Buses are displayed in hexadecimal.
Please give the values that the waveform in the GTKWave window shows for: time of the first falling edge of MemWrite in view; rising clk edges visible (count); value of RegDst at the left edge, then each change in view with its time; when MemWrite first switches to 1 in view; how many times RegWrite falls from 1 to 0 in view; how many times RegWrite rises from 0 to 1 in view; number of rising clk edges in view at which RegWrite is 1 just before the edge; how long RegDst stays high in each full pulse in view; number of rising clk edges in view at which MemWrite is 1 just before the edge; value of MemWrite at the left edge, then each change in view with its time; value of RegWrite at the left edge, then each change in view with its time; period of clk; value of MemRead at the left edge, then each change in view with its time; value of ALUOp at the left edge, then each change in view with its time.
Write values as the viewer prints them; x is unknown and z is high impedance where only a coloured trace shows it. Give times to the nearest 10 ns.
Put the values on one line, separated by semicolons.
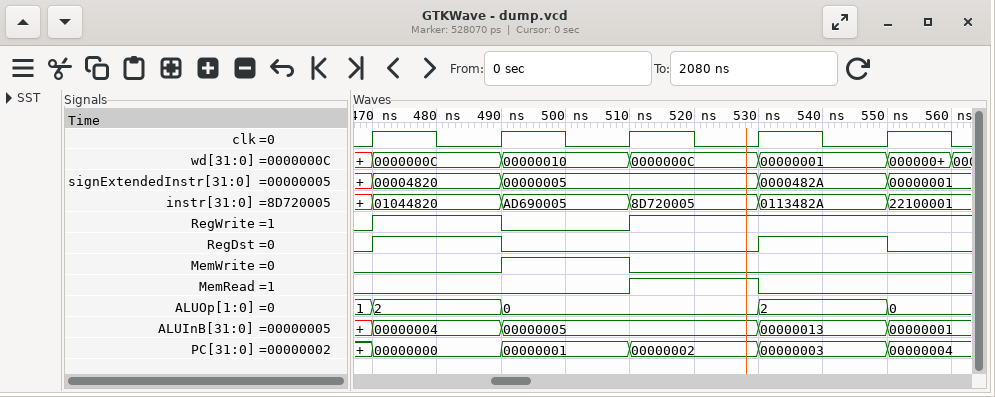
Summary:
510 ns; 5; 0, 1 at 470 ns, 0 at 490 ns, 1 at 530 ns, 0 at 550 ns; 490 ns; 1; 2; 3; 20 ns, 20 ns; 1; 0, 1 at 490 ns, 0 at 510 ns; 0, 1 at 470 ns, 0 at 490 ns, 1 at 510 ns; 20 ns; 0, 1 at 510 ns, 0 at 530 ns; 1, 2 at 470 ns, 0 at 490 ns, 2 at 530 ns, 0 at 550 ns
